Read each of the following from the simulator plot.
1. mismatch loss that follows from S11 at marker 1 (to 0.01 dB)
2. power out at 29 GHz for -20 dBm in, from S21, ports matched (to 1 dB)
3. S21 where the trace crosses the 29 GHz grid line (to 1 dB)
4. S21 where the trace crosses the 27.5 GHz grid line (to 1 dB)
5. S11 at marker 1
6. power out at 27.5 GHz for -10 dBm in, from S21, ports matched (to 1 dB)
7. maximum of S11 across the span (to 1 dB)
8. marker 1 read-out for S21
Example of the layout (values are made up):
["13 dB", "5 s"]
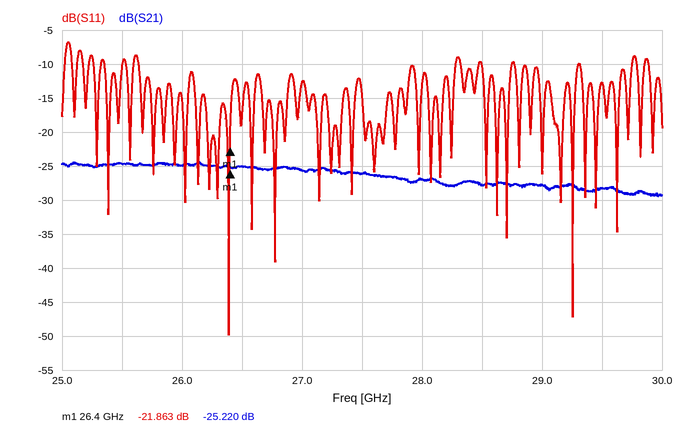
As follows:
["0.03 dB", "-48 dBm", "-28 dB", "-26 dB", "-21.863 dB", "-36 dBm", "-7 dB", "-25.220 dB"]
